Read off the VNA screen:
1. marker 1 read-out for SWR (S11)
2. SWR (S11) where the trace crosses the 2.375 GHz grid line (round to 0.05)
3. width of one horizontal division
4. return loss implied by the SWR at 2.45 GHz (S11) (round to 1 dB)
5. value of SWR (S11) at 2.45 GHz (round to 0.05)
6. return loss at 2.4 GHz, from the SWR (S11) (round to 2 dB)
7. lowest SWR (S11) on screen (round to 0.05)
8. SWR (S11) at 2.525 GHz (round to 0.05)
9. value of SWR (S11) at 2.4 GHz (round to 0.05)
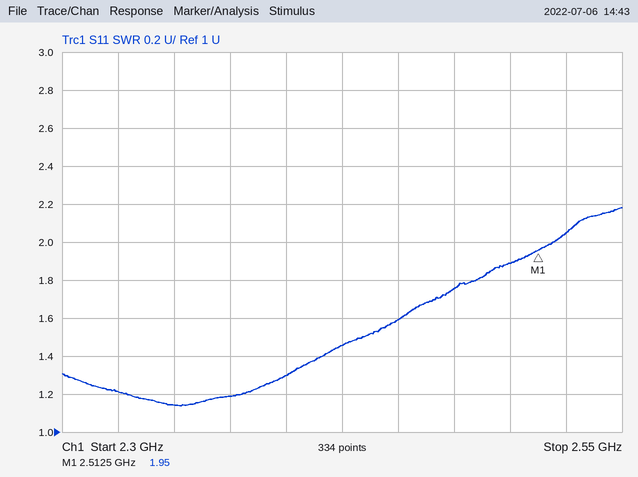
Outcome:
1.95
1.20
25 MHz
13 dB
1.60
18 dB
1.15
2.05
1.30
